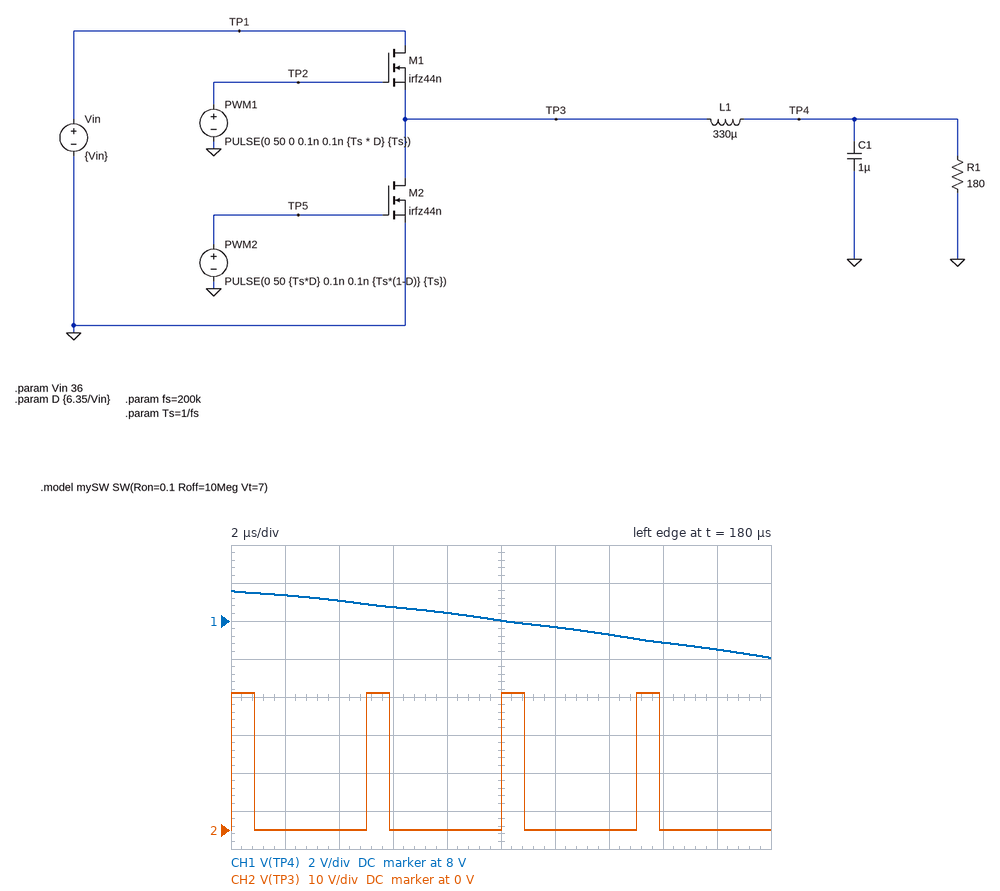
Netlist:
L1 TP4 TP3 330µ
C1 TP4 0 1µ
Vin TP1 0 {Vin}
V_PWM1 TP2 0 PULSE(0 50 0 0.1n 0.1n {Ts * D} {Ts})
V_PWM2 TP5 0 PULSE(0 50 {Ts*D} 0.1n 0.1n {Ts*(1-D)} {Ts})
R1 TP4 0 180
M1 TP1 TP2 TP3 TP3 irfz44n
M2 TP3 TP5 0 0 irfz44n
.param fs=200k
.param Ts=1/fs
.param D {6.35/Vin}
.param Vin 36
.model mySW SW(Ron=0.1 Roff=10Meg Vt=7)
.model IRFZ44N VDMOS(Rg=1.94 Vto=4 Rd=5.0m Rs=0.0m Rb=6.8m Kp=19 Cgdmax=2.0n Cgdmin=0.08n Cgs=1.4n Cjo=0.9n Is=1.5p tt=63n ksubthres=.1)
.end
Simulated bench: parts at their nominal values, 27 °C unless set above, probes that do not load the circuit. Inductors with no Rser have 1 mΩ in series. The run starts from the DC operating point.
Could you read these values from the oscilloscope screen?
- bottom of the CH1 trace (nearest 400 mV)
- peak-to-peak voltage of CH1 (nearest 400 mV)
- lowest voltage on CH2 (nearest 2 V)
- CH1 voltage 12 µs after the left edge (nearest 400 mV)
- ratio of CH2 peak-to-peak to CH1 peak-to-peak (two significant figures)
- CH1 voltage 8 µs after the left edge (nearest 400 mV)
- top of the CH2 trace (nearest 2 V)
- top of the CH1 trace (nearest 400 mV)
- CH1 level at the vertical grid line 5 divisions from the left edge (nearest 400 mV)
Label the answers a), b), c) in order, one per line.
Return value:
a) 6.0 V
b) 3.6 V
c) 0 V
d) 7.6 V
e) 10
f) 8.4 V
g) 36 V
h) 9.6 V
i) 8.0 V
